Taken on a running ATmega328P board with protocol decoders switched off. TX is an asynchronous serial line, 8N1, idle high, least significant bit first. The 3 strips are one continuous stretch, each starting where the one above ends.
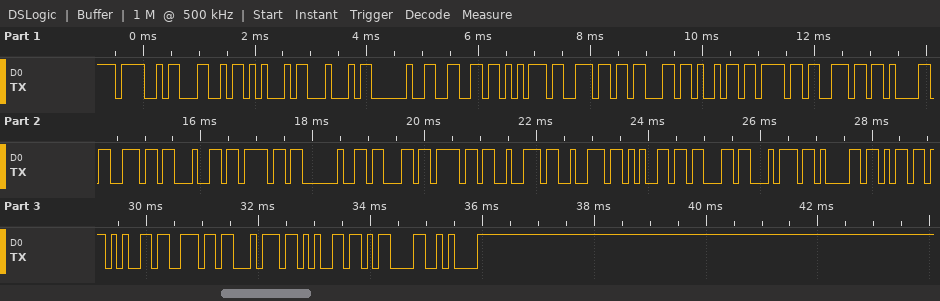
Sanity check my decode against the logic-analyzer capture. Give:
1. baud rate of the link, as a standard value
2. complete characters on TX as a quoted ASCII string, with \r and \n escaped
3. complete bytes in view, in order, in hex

9600 baud
"OLED funcionando correctamente\r\n"
4F 4C 45 44 20 66 75 6E 63 69 6F 6E 61 6E 64 6F 20 63 6F 72 72 65 63 74 61 6D 65 6E 74 65 0D 0A
